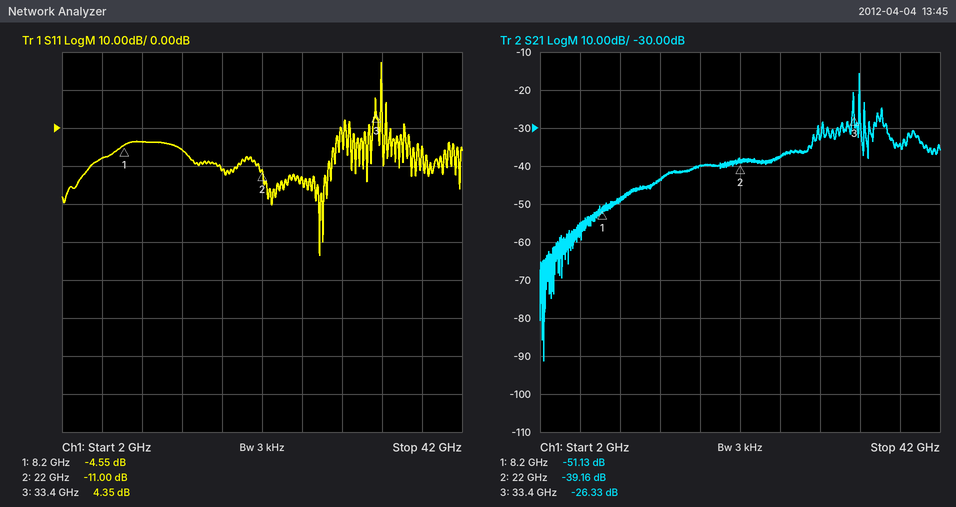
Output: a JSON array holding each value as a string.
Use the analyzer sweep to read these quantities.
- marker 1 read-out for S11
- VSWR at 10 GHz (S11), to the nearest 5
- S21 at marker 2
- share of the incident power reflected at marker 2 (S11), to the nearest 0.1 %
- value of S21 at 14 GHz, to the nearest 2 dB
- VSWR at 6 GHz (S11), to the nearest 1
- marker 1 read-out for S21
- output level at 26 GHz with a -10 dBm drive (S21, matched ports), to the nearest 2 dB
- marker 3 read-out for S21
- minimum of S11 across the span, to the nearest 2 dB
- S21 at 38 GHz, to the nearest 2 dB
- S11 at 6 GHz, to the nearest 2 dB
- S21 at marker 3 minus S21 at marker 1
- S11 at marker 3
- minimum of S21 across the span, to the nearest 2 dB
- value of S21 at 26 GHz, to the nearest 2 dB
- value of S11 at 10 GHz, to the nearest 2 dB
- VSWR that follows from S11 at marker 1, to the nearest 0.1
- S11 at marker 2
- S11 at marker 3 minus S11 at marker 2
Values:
["-4.55 dB", "5", "-39.16 dB", "7.9 %", "-44 dB", "2", "-51.13 dB", "-48 dBm", "-26.33 dB", "-34 dB", "-34 dB", "-8 dB", "24.80 dB", "4.35 dB", "-92 dB", "-38 dB", "-4 dB", "3.9", "-11.00 dB", "15.35 dB"]
